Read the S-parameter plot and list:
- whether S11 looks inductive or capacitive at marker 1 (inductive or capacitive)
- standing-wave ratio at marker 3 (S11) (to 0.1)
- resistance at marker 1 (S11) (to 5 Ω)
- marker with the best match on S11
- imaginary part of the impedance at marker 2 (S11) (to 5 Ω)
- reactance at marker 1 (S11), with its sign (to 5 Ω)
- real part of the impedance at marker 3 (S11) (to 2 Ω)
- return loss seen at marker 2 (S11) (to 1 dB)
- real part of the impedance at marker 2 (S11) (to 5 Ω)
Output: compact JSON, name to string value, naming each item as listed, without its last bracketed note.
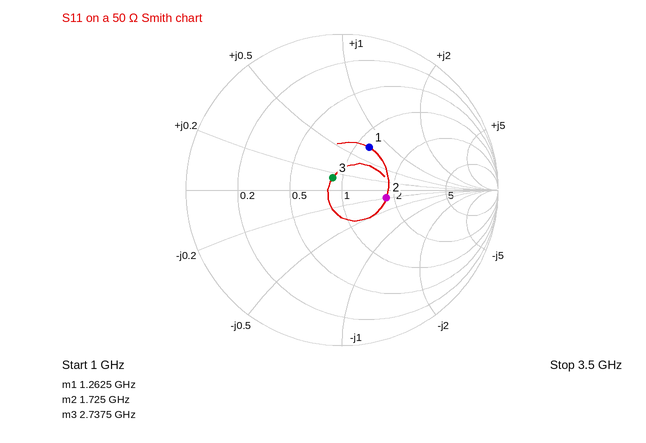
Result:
{"whether S11 looks inductive or capacitive at marker 1": "inductive", "standing-wave ratio at marker 3 (S11)": "1.2", "resistance at marker 1 (S11)": "60 Ω", "marker with the best match on S11": "marker 3", "imaginary part of the impedance at marker 2 (S11)": "-10 Ω", "reactance at marker 1 (S11), with its sign": "+35 Ω", "real part of the impedance at marker 3 (S11)": "44 Ω", "return loss seen at marker 2 (S11)": "11 dB", "real part of the impedance at marker 2 (S11)": "90 Ω"}
